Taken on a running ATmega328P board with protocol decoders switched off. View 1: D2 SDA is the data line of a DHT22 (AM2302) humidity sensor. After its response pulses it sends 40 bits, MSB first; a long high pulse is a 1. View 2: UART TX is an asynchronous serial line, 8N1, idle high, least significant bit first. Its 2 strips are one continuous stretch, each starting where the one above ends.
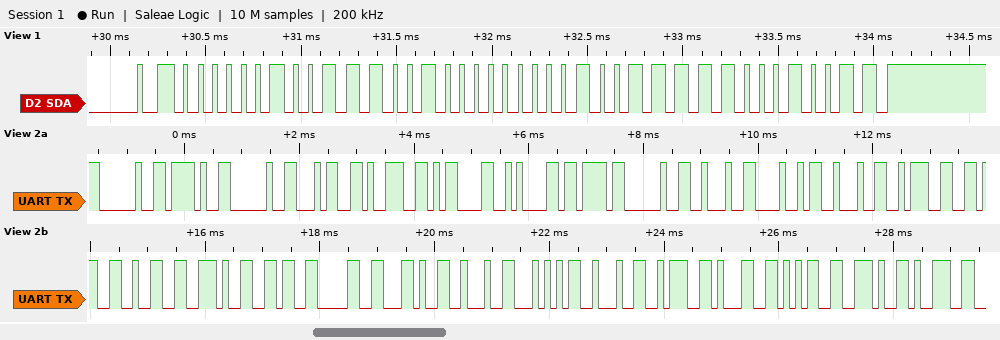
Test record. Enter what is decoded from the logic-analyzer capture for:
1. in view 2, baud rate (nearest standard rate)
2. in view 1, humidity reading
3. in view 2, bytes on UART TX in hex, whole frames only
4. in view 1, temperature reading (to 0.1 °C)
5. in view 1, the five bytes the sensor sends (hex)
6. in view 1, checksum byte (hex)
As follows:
9600 baud
62.6 %
20 2F 20 34 39 0D 0A 7B 20 22 48 22 3A 36 32 2E 36 30 2C 22 54 22 3A 31 35 2E 39
15.9 °C
02 72 00 9F 13
0x13
